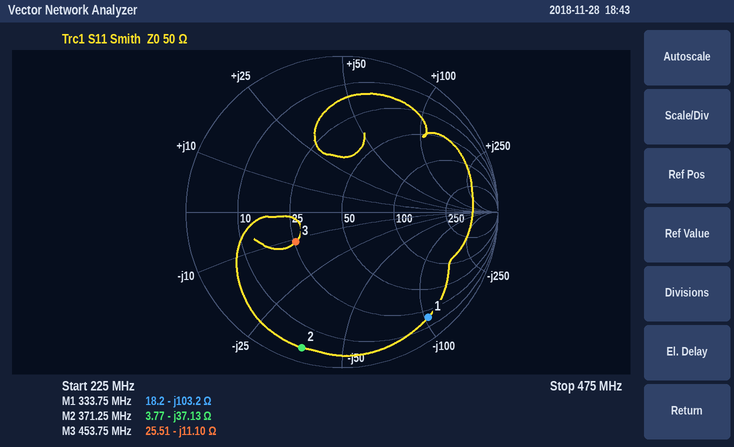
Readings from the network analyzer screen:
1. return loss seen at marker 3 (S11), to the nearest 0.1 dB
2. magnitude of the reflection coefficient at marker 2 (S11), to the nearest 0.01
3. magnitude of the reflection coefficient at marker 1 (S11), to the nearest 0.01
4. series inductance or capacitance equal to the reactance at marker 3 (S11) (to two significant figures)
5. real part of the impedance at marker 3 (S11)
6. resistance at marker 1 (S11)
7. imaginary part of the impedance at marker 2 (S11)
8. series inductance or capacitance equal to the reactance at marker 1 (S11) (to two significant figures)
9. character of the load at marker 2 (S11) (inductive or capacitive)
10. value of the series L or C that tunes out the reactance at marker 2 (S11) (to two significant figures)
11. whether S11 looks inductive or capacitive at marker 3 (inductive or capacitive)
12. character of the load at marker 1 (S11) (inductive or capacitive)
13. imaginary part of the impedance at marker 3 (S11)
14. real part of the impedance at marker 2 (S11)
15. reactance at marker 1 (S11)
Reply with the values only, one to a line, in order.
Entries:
9.1 dB
0.91
0.87
32 pF
25.51 Ω
18.2 Ω
-37.13 Ω
4.6 pF
capacitive
16 nH
capacitive
capacitive
-11.10 Ω
3.77 Ω
-103.2 Ω
